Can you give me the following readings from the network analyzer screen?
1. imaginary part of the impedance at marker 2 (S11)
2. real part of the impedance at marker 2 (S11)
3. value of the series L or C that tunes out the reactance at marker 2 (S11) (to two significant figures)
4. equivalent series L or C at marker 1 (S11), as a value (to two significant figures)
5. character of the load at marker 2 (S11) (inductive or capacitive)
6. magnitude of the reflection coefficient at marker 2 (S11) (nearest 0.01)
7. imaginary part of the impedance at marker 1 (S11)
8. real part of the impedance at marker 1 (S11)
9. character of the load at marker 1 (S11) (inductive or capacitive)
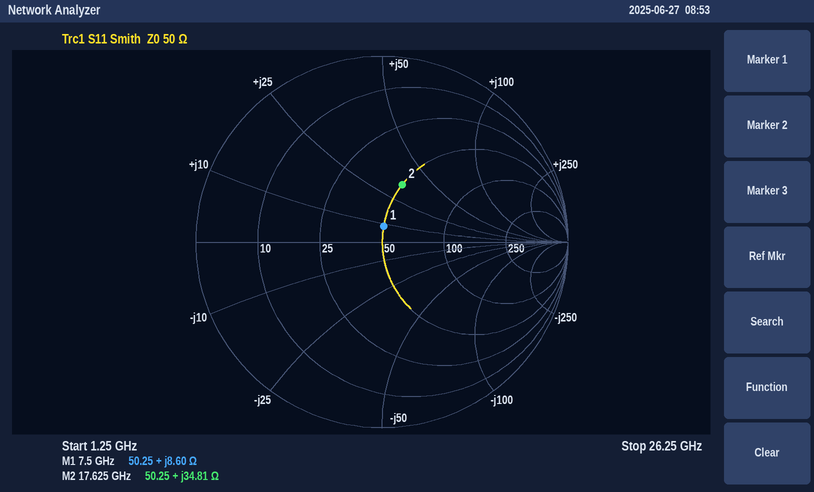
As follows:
+34.81 Ω
50.25 Ω
260 fF
180 pH
inductive
0.33
+8.60 Ω
50.25 Ω
inductive
